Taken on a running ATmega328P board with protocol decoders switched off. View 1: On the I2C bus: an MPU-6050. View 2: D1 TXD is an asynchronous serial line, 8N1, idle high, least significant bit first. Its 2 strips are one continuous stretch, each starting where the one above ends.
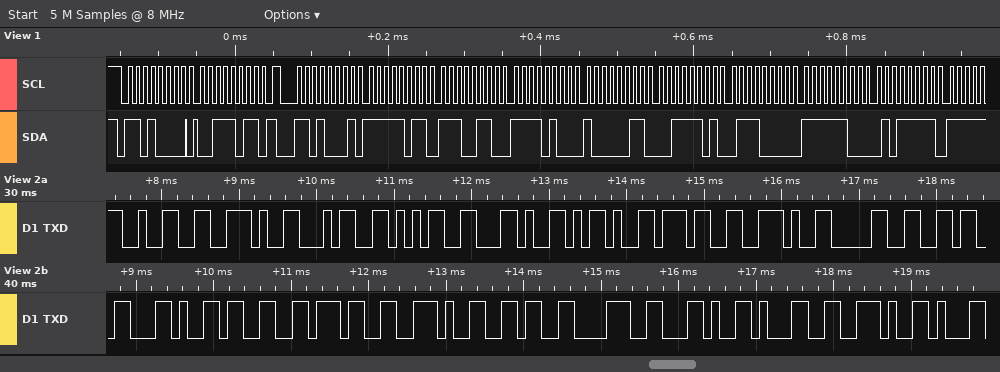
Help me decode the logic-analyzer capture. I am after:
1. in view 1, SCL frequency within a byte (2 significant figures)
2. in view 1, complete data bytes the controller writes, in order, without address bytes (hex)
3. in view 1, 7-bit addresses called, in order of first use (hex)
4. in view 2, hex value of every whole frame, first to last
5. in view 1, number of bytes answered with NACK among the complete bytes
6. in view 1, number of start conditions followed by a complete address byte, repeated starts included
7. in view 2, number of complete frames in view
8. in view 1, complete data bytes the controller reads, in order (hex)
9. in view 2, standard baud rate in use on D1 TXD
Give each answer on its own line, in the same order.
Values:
100 kHz
3B
0x68
32 2E 34 35 2C 2D 37 2E 30 36 2C 33 37 2E 36 38 2C 31 2E
0
2
19
FB E6 F4 83 3D 70 FC 5F
9600 baud
